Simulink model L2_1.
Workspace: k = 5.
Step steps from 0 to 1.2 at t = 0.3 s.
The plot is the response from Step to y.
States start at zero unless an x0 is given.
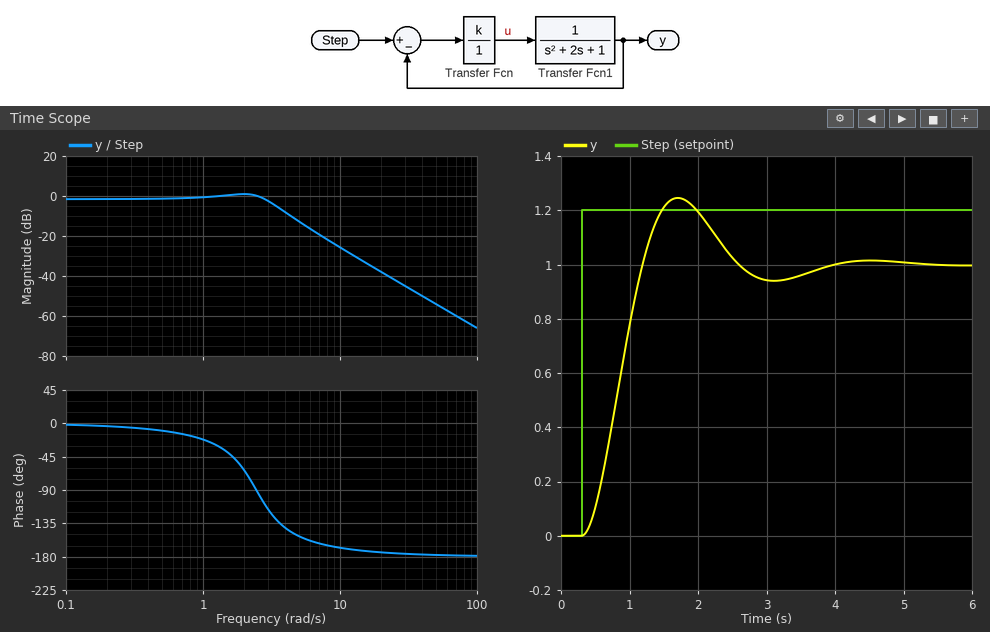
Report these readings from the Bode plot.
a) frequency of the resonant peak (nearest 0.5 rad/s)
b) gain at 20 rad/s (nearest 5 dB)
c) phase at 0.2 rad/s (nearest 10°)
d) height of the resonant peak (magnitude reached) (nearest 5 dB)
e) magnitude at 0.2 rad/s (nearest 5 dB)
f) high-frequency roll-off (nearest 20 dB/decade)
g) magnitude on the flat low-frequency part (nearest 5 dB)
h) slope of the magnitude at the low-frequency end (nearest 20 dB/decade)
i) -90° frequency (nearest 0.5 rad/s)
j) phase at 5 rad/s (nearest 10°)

2.0 rad/s
-40 dB
0°
0 dB
0 dB
-40 dB/decade
0 dB
0 dB/decade
2.5 rad/s
-150°
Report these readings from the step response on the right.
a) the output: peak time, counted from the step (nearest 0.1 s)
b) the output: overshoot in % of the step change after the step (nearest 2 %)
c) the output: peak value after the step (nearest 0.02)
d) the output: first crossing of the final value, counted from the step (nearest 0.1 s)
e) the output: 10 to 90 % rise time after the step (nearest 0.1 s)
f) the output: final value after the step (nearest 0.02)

1.4 s
24 %
1.24
0.9 s
0.6 s
1.00
